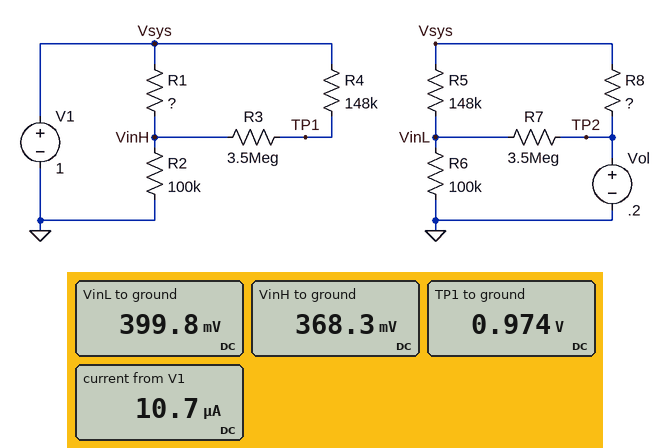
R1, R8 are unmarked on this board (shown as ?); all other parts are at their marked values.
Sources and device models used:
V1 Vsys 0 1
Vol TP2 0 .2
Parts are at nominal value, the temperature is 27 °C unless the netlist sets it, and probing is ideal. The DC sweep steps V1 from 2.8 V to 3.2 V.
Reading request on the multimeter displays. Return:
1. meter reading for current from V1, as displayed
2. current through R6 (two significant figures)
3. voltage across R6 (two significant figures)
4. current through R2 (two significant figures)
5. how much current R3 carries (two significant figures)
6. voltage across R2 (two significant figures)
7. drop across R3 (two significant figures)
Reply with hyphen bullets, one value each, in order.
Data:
- 10.7 µA
- 4.0 µA
- 400 mV
- 3.7 µA
- 170 nA
- 370 mV
- 610 mV
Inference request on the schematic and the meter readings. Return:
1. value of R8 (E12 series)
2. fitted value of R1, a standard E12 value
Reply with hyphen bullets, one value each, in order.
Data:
- 270 kΩ
- 180 kΩ
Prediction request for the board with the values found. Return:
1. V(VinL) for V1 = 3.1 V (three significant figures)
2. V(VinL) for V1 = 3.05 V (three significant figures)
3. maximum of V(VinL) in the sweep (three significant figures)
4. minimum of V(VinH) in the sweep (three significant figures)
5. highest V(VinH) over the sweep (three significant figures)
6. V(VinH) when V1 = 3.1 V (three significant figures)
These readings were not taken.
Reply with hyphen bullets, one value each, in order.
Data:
- 1.23 V
- 1.21 V
- 1.27 V
- 1.03 V
- 1.18 V
- 1.14 V
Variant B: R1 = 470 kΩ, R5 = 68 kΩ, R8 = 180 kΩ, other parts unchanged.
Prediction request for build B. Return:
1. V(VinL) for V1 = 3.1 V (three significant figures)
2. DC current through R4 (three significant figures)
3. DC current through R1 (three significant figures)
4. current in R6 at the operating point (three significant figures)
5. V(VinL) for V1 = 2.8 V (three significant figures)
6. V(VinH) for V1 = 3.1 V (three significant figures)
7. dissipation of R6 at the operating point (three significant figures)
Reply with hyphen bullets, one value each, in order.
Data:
- 1.83 V
- 221 nA
- 1.72 µA
- 5.91 µA
- 1.65 V
- 600 mV
- 3.49 µW
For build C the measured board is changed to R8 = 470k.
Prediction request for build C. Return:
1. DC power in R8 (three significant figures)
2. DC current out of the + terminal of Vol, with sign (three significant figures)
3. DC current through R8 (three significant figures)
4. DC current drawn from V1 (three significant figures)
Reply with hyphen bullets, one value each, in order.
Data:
- 1.36 µW
- -1.76 µA
- 1.70 µA
- 9.44 µA
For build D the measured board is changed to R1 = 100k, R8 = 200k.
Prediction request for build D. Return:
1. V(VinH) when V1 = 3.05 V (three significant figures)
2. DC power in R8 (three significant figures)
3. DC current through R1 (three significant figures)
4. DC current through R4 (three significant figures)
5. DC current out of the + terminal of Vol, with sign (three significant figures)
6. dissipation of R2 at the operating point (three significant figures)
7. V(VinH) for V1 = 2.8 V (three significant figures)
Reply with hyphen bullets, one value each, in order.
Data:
- 1.55 V
- 3.20 µW
- 4.93 µA
- 135 nA
- -4.06 µA
- 2.57 µW
- 1.42 V
